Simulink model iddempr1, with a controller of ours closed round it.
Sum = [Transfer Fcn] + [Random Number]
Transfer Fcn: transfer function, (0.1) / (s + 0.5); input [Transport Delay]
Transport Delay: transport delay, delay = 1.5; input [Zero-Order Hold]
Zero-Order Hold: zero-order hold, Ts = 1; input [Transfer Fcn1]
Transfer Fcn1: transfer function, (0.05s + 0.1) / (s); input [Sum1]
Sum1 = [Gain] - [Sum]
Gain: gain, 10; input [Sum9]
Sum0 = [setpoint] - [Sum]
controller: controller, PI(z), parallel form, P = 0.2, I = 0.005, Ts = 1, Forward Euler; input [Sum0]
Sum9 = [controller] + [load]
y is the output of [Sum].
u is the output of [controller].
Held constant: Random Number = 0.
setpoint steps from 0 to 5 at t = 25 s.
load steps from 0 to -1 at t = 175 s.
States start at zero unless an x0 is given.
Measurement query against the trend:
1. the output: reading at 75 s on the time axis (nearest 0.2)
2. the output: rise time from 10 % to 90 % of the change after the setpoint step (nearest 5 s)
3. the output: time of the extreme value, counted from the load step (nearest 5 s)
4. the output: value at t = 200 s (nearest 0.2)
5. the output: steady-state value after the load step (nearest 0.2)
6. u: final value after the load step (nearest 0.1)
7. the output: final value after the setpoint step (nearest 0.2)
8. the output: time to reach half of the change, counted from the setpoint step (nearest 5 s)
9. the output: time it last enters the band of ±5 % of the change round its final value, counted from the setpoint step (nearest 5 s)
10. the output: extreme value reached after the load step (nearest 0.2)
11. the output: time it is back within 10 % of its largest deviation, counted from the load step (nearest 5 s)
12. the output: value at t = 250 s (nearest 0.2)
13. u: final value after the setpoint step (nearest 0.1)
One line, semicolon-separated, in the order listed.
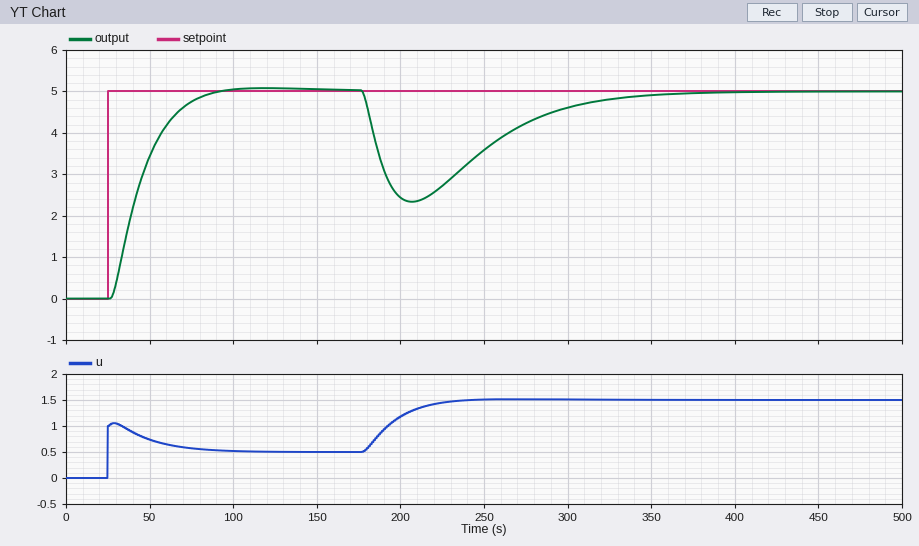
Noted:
4.8; 35 s; 30 s; 2.4; 5.0; 1.5; 5.0; 15 s; 50 s; 2.4; 140 s; 3.6; 0.5
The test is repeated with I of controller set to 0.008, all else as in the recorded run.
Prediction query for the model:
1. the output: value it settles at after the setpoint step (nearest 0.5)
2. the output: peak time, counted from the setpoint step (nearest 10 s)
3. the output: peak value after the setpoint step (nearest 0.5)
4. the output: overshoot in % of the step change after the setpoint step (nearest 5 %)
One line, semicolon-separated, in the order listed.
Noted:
5.0; 60 s; 5.5; 10 %
